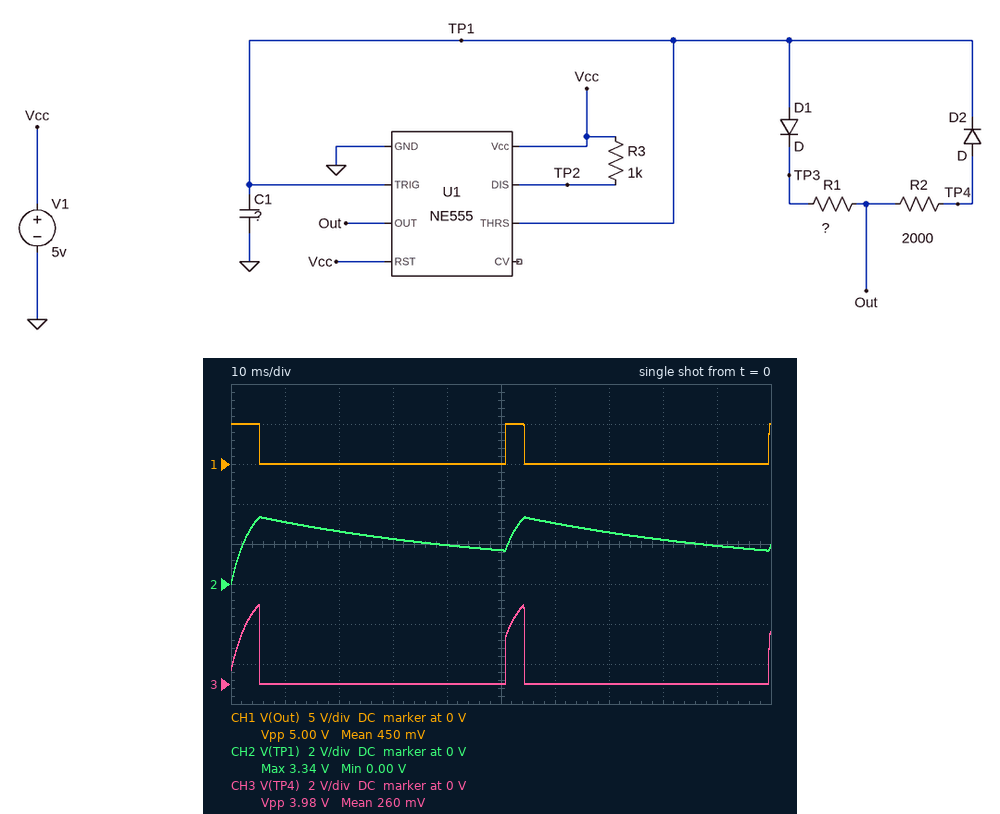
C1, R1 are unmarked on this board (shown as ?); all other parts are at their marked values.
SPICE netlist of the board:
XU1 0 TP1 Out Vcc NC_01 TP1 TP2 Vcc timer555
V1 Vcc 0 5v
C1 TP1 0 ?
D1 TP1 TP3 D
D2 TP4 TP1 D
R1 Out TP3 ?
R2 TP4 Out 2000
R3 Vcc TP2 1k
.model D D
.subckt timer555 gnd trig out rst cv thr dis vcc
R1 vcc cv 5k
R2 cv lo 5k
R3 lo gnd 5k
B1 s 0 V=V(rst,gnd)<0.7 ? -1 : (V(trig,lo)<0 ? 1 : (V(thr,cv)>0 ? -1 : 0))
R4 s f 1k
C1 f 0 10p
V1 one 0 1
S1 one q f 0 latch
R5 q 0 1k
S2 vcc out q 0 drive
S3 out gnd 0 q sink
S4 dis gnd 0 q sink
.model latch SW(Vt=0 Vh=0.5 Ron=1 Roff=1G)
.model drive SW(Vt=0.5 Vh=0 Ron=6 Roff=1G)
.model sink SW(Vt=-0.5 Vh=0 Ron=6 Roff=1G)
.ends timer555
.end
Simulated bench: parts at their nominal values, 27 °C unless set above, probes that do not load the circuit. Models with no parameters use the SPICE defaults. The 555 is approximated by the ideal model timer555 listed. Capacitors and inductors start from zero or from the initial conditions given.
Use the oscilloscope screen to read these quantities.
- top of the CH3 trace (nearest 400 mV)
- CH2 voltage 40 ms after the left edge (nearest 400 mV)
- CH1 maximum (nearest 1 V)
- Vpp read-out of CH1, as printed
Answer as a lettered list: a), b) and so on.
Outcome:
a) 4.0 V
b) 2.0 V
c) 5 V
d) 5.00 V
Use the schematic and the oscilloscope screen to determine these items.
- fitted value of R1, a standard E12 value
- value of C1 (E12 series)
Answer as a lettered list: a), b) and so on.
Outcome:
a) 27 kΩ
b) 1.8 µF
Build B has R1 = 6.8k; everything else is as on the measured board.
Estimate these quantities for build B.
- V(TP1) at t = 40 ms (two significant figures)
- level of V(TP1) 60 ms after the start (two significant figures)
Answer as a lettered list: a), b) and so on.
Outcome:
a) 2.5 V
b) 1.9 V
